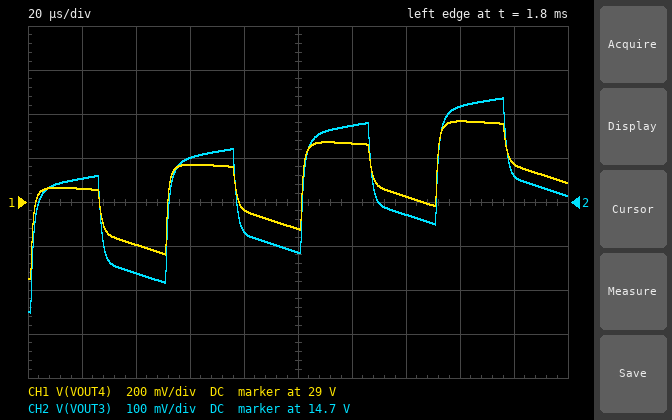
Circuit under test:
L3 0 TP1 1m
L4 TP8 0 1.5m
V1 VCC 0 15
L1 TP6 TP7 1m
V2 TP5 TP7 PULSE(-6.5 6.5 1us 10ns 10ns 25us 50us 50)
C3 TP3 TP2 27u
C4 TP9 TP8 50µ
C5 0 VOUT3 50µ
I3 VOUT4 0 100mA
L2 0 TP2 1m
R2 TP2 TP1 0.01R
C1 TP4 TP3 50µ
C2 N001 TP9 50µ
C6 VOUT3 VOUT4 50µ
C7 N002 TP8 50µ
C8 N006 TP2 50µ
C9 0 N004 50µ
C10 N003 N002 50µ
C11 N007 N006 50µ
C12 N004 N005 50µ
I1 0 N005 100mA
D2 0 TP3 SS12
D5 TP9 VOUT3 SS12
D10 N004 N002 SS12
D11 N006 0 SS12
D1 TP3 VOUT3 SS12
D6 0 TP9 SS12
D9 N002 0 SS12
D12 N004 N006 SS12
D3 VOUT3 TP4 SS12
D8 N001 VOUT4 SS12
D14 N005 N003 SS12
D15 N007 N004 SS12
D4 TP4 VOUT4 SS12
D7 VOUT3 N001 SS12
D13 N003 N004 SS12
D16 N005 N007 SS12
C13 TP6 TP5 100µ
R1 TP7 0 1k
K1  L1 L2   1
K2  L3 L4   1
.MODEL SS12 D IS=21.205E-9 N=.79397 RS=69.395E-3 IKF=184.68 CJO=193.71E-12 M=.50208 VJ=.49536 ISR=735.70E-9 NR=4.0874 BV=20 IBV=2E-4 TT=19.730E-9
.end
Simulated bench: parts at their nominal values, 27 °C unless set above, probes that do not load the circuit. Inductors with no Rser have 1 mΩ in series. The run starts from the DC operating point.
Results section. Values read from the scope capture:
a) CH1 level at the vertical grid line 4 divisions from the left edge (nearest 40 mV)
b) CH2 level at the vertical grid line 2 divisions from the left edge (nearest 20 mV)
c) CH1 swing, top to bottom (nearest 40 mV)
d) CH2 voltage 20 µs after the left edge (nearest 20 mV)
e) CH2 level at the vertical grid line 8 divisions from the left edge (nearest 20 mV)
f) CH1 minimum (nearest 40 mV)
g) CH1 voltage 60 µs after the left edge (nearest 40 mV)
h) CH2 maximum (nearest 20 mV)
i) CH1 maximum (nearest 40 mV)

28.96 V
14.54 V
720 mV
14.76 V
14.92 V
28.64 V
29.16 V
14.94 V
29.36 V
